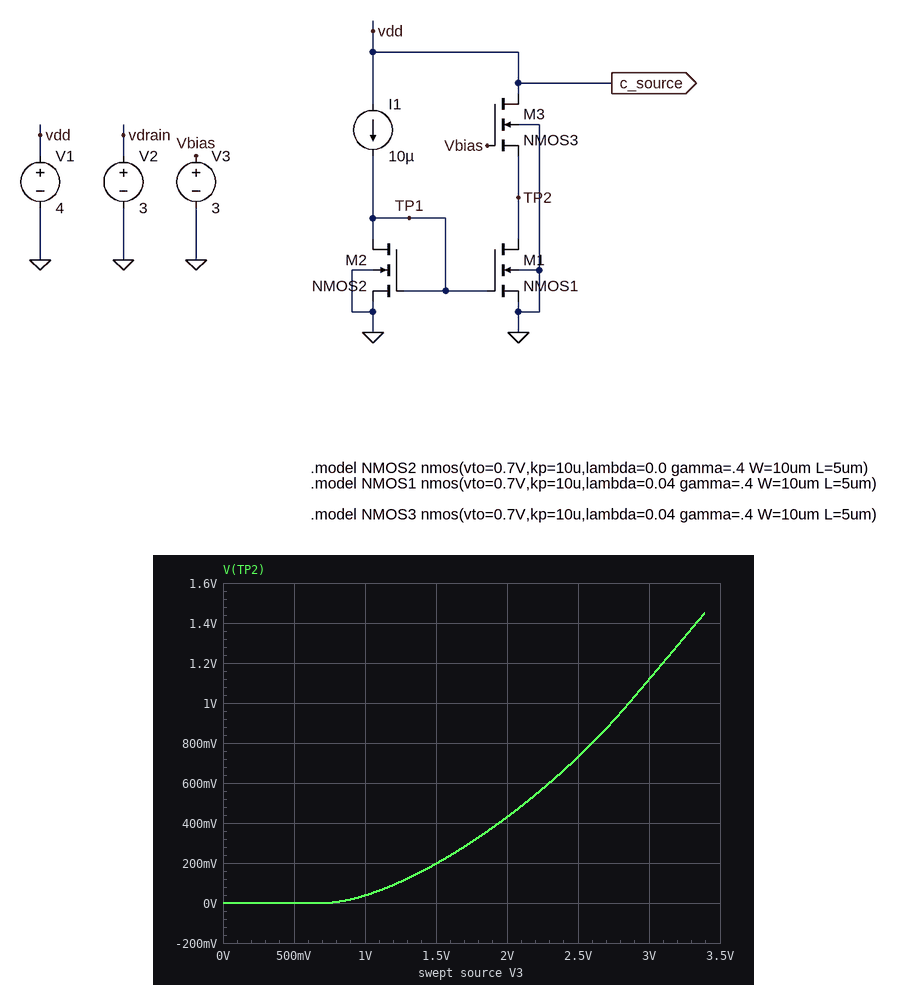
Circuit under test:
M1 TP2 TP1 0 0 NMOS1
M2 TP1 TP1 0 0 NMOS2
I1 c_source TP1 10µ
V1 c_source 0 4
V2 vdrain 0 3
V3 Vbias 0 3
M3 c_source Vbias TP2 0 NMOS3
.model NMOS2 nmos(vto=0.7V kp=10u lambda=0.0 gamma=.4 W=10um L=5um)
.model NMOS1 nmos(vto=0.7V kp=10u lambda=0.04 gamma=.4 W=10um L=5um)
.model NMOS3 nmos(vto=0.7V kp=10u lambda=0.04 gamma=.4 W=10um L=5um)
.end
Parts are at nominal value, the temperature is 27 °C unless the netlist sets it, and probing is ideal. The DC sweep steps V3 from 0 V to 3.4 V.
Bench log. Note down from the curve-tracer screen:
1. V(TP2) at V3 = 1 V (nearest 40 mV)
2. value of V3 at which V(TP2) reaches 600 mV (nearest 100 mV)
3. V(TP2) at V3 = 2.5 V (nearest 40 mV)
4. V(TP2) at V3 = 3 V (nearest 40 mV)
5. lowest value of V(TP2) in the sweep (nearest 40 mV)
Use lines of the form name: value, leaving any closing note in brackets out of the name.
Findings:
V(TP2) at V3 = 1 V: 40 mV
value of V3 at which V(TP2) reaches 600 mV: 2.3 V
V(TP2) at V3 = 2.5 V: 720 mV
V(TP2) at V3 = 3 V: 1.12 V
lowest value of V(TP2) in the sweep: 0 V
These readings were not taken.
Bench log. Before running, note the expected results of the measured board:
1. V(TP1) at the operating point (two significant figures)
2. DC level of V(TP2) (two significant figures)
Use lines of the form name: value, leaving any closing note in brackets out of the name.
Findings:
V(TP1) at the operating point: 1.7 V
DC level of V(TP2): 1.1 V
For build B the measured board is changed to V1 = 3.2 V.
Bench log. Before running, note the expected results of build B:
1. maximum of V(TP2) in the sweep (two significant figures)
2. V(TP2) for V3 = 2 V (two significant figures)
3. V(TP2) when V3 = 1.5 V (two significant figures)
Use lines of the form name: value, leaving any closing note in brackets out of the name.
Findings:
maximum of V(TP2) in the sweep: 1.4 V
V(TP2) for V3 = 2 V: 420 mV
V(TP2) when V3 = 1.5 V: 190 mV
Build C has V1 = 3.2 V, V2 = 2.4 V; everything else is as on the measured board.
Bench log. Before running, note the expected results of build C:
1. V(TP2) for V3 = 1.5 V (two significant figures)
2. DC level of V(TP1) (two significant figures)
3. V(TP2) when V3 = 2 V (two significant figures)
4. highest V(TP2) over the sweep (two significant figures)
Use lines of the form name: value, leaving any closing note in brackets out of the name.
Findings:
V(TP2) for V3 = 1.5 V: 190 mV
DC level of V(TP1): 1.7 V
V(TP2) when V3 = 2 V: 420 mV
highest V(TP2) over the sweep: 1.4 V
